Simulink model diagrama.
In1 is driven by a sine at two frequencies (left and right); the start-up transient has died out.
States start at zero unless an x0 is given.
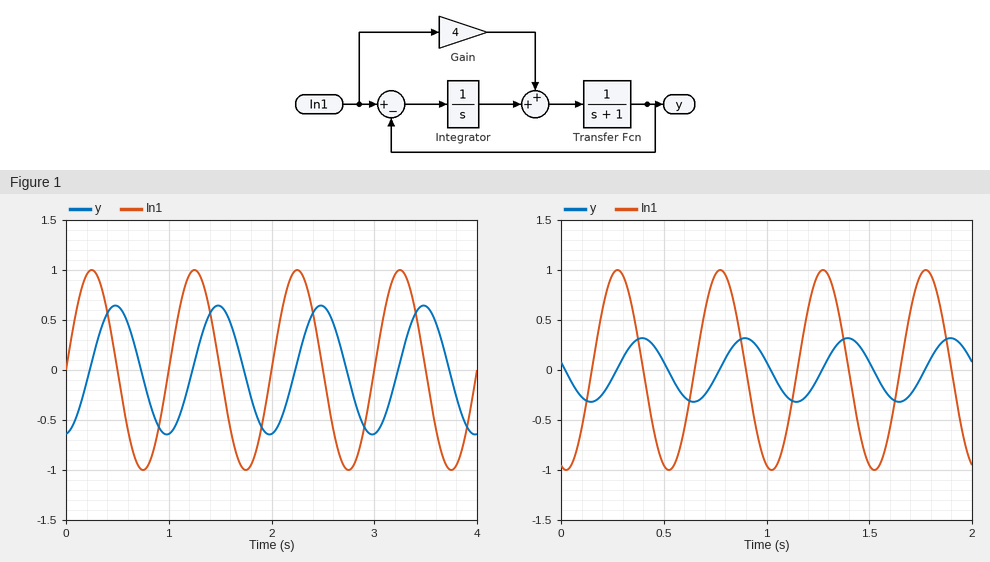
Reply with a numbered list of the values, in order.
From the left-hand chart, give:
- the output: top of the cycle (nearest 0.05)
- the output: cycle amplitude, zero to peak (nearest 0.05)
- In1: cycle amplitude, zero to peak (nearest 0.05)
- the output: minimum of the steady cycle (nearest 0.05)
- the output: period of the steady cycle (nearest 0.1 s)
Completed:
1. 0.65
2. 0.65
3. 1.00
4. -0.65
5. 1.0 s
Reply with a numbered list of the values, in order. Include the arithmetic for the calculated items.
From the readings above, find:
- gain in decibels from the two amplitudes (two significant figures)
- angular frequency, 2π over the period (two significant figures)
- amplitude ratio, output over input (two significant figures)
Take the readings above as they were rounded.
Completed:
1. 20 log10(0.65 / 1) = -3.7 dB
2. 2π / 1 = 6.3 rad/s
3. 0.65 / 1 = 0.65
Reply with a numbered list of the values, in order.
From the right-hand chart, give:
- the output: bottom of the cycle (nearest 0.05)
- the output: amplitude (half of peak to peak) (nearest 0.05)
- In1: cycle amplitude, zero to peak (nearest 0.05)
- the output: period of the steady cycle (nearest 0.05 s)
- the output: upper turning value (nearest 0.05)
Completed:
1. -0.30
2. 0.30
3. 1.00
4. 0.50 s
5. 0.30
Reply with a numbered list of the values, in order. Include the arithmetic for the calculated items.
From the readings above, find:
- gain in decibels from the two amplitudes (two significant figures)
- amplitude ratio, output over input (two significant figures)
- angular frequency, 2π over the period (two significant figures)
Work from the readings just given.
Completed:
1. 20 log10(0.3 / 1) = -10 dB
2. 0.3 / 1 = 0.30
3. 2π / 0.5 = 13 rad/s
